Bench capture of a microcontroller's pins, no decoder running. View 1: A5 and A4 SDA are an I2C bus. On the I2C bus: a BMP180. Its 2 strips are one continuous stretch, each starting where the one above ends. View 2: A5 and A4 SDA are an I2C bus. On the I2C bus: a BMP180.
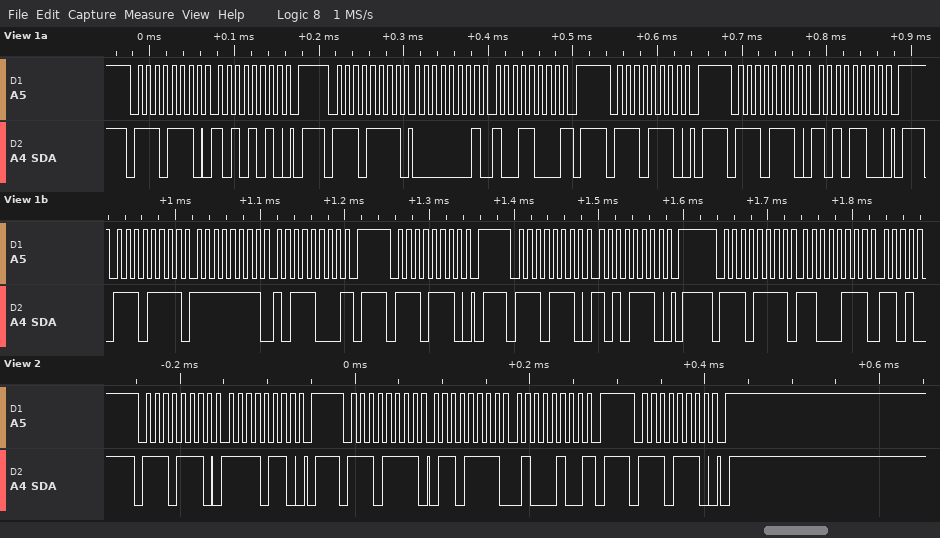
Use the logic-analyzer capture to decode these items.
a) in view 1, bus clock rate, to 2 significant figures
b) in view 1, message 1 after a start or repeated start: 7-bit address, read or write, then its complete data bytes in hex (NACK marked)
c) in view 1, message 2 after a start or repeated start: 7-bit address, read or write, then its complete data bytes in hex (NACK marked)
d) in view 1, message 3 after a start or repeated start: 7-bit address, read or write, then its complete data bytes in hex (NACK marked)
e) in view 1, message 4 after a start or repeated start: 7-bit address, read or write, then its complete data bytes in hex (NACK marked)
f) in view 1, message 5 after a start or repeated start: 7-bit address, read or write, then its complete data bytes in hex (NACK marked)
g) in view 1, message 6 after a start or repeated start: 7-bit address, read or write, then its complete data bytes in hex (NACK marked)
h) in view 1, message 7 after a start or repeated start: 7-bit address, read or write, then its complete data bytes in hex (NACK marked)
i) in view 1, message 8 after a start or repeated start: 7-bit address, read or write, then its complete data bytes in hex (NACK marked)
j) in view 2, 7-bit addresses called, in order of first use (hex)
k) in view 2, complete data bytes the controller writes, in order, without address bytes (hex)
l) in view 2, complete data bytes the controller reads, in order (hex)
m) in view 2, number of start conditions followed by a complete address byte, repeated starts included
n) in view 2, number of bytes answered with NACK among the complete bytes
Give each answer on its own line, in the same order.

100 kHz
0x77 write: AA
0x77 read: 01 98 NACK
0x77 write
0x77 write: AC
0x77 read: FF B8 NACK
0x77 write
0x77 write: AE
0x77 read: C7
0x77
F6
6F 44
3
1
